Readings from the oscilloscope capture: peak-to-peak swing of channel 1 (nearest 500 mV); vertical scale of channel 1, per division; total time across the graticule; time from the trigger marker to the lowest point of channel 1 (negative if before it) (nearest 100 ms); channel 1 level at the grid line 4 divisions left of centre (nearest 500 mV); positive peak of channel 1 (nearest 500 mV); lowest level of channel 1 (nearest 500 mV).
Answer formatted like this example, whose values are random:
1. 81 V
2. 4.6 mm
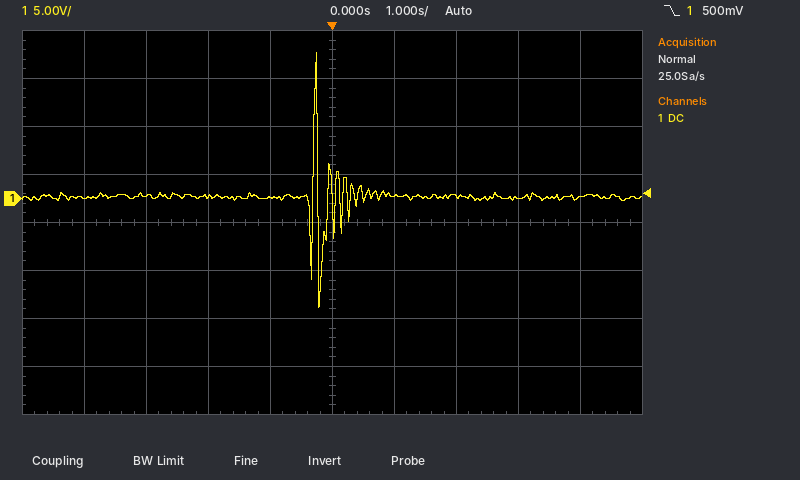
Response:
1. 26.5 V
2. 5 V
3. 10 s
4. -200 ms
5. 0.0 V
6. 15.0 V
7. -11.5 V
